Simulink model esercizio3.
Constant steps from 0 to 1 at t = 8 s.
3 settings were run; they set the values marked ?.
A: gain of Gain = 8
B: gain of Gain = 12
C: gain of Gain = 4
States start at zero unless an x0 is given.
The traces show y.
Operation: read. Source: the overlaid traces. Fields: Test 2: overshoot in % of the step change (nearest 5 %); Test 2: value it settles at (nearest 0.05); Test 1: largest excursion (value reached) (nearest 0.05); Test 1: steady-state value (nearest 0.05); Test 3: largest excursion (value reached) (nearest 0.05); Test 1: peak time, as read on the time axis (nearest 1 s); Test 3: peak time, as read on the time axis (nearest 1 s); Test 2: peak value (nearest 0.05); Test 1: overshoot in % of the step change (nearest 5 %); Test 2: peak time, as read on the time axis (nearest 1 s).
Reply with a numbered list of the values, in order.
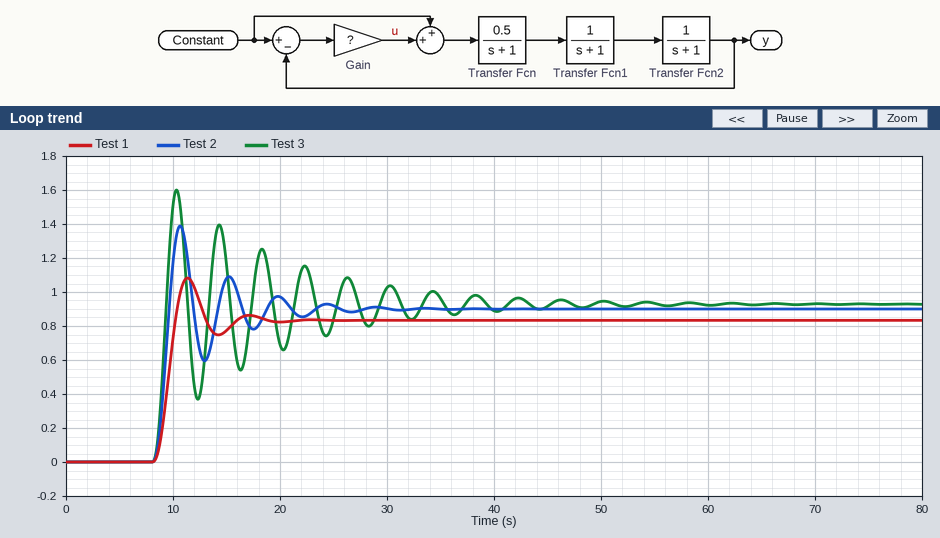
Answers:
1. 55 %
2. 0.90
3. 1.10
4. 0.85
5. 1.60
6. 11 s
7. 10 s
8. 1.40
9. 30 %
10. 11 s
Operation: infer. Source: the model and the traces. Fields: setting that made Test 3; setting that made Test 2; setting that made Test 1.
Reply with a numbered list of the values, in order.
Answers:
1. B
2. A
3. C
